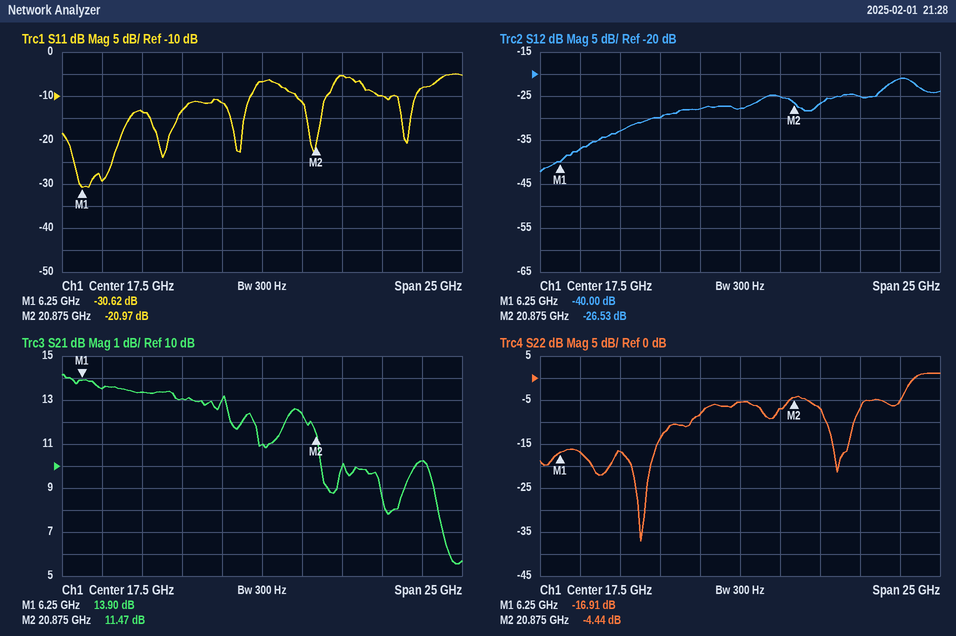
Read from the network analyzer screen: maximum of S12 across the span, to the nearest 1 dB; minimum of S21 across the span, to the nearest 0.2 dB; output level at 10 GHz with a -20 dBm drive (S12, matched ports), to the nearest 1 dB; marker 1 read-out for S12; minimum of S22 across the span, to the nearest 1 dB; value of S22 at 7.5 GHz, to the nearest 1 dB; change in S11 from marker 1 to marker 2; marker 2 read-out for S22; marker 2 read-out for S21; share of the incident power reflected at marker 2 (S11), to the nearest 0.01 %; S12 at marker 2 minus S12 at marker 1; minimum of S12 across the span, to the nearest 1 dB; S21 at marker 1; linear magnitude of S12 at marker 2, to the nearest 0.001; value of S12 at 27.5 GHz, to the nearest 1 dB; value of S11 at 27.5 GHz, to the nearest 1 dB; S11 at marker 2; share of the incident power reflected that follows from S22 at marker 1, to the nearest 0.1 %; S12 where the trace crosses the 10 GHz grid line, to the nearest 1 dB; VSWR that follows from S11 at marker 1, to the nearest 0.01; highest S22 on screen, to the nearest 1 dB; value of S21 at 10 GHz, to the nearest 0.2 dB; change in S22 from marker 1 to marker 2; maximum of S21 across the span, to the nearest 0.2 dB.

-21 dB
5.6 dB
-53 dBm
-40.00 dB
-37 dB
-17 dB
9.65 dB
-4.44 dB
11.47 dB
0.80 %
13.47 dB
-42 dB
13.90 dB
0.047
-21 dB
-8 dB
-20.97 dB
2.0 %
-33 dB
1.06
1 dB
13.4 dB
12.47 dB
14.2 dB
